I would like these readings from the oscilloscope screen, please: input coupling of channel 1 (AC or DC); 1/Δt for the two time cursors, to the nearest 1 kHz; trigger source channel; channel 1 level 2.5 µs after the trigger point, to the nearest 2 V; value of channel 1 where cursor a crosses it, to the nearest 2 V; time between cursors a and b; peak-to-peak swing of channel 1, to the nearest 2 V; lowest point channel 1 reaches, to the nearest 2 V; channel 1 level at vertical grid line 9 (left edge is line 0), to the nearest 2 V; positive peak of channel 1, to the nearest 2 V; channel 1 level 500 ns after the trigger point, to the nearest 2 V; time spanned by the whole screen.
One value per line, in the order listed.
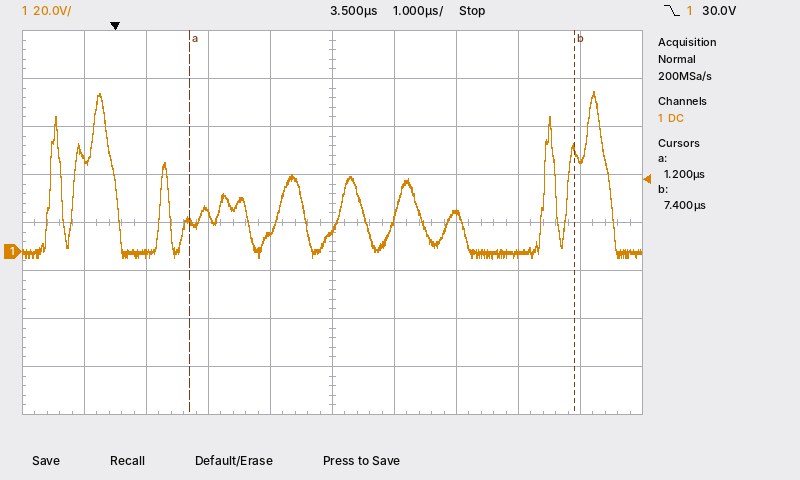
DC
161 kHz
channel 1
8 V
12 V
6.2 µs
70 V
-4 V
38 V
66 V
0 V
10 µs
